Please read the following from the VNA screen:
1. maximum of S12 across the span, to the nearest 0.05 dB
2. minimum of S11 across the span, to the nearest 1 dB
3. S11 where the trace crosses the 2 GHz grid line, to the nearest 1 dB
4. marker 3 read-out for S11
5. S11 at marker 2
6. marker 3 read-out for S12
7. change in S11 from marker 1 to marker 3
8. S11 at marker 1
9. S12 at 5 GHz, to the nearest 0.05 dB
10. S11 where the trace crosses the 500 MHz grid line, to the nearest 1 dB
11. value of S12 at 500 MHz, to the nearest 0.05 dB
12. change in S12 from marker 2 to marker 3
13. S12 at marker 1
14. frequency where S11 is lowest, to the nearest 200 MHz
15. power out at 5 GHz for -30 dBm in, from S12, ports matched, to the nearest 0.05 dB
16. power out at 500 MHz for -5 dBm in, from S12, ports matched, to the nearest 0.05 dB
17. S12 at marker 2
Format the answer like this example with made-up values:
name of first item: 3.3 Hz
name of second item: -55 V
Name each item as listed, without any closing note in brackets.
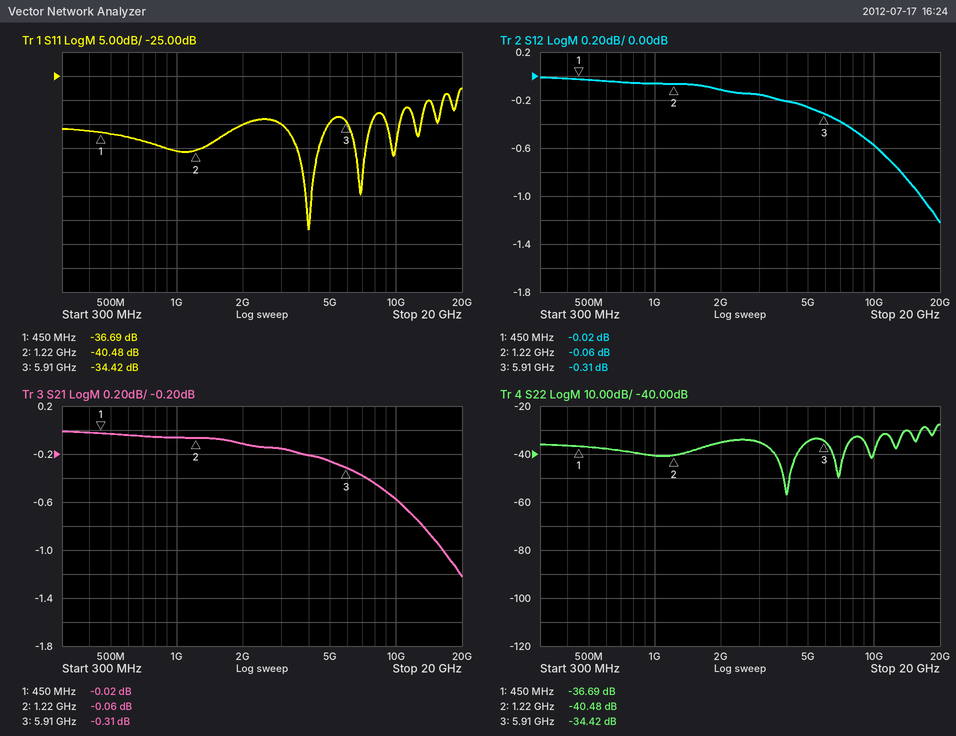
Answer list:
maximum of S12 across the span, to the nearest 0.05 dB: 0.00 dB
minimum of S11 across the span, to the nearest 1 dB: -57 dB
S11 where the trace crosses the 2 GHz grid line, to the nearest 1 dB: -35 dB
marker 3 read-out for S11: -34.42 dB
S11 at marker 2: -40.48 dB
marker 3 read-out for S12: -0.31 dB
change in S11 from marker 1 to marker 3: 2.27 dB
S11 at marker 1: -36.69 dB
S12 at 5 GHz, to the nearest 0.05 dB: -0.25 dB
S11 where the trace crosses the 500 MHz grid line, to the nearest 1 dB: -37 dB
value of S12 at 500 MHz, to the nearest 0.05 dB: -0.05 dB
change in S12 from marker 2 to marker 3: -0.25 dB
S12 at marker 1: -0.02 dB
frequency where S11 is lowest, to the nearest 200 MHz: 4.0 GHz
power out at 5 GHz for -30 dBm in, from S12, ports matched, to the nearest 0.05 dB: -30.25 dBm
power out at 500 MHz for -5 dBm in, from S12, ports matched, to the nearest 0.05 dB: -5.05 dBm
S12 at marker 2: -0.06 dB
